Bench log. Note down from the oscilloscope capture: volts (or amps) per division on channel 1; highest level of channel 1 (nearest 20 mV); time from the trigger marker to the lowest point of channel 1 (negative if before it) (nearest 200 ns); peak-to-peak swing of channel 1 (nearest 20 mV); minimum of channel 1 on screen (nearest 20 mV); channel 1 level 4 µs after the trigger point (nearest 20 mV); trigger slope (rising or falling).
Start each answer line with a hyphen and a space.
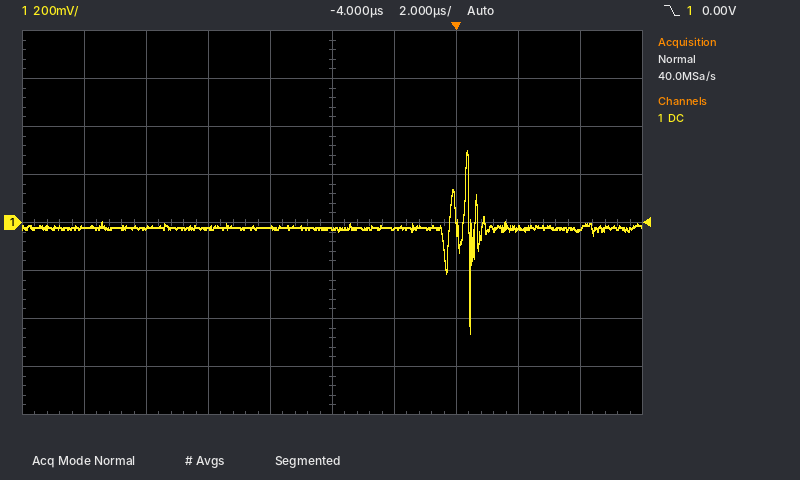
- 200 mV
- 300 mV
- +400 ns
- 760 mV
- -460 mV
- -20 mV
- falling
